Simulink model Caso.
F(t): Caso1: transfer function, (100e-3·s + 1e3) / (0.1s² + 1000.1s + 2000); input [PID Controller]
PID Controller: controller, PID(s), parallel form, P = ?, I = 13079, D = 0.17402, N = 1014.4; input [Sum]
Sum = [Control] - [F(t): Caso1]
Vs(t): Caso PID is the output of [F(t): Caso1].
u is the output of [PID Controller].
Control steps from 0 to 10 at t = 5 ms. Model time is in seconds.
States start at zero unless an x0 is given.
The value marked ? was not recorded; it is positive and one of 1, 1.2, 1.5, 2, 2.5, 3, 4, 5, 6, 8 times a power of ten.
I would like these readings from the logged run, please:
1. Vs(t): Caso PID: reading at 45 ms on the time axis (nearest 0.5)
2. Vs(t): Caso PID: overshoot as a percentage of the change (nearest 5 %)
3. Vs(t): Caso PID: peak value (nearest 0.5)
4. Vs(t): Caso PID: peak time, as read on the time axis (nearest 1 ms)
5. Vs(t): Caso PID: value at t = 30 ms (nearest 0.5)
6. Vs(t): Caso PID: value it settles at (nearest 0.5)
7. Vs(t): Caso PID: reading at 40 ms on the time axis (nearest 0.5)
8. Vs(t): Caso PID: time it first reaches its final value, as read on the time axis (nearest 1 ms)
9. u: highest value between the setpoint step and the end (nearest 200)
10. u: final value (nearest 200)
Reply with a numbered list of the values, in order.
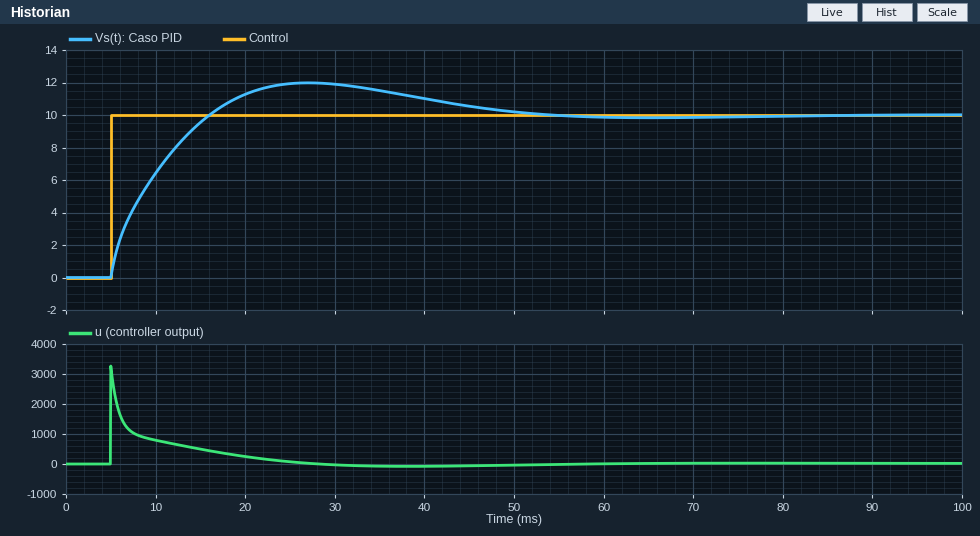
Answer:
1. 10.5
2. 20 %
3. 12.0
4. 27 ms
5. 12.0
6. 10.0
7. 11.0
8. 16 ms
9. 3200
10. 0
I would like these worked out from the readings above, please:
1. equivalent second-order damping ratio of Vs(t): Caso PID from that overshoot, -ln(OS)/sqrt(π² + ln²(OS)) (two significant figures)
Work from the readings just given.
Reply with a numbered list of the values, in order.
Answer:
1. 0.46
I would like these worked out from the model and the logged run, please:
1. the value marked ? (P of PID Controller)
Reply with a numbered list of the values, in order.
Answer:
1. 150
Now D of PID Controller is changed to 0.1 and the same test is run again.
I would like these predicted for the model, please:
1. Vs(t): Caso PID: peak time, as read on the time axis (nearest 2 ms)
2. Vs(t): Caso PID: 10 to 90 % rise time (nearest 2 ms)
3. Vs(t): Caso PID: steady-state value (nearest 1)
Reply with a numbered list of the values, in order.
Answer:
1. 26 ms
2. 8 ms
3. 10
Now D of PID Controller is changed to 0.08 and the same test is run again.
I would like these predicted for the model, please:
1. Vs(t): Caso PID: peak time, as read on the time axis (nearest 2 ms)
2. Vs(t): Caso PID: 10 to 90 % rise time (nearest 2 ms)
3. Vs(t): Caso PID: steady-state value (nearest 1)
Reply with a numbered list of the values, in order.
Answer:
1. 26 ms
2. 8 ms
3. 10
